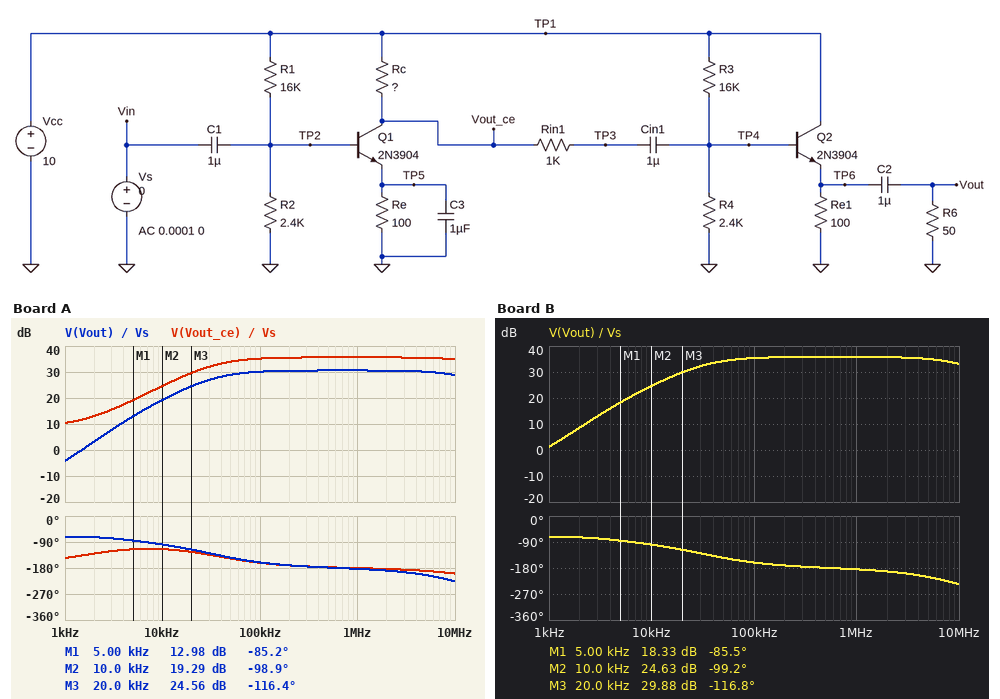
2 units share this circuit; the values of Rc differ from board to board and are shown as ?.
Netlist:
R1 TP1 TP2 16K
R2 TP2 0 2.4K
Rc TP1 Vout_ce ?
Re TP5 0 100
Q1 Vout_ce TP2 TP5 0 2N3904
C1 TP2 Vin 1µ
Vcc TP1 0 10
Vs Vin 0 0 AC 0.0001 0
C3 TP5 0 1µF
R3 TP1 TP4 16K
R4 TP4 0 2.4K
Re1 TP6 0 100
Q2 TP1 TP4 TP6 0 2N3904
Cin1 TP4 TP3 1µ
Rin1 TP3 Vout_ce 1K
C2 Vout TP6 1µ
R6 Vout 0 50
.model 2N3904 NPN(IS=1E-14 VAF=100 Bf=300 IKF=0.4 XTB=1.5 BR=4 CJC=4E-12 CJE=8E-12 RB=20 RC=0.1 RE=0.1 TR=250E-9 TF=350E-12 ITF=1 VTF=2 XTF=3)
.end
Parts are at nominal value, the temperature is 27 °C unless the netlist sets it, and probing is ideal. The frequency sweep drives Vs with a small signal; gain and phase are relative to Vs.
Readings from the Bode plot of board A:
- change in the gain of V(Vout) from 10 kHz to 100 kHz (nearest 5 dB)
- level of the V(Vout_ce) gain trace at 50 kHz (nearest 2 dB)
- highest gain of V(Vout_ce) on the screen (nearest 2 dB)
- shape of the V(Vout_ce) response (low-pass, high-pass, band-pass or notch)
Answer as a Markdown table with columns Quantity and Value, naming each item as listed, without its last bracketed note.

| Quantity | Value |
|---|---|
| change in the gain of V(Vout) from 10 kHz to 100 kHz | 10 dB |
| level of the V(Vout_ce) gain trace at 50 kHz | 34 dB |
| highest gain of V(Vout_ce) on the screen | 36 dB |
| shape of the V(Vout_ce) response | high-pass |
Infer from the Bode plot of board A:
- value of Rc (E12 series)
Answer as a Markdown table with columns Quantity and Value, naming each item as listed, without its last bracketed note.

| Quantity | Value |
|---|---|
| value of Rc | 330 Ω |
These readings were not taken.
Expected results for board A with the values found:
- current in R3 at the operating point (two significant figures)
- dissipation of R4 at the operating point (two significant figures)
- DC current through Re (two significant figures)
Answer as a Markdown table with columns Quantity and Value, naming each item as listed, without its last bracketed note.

| Quantity | Value |
|---|---|
| current in R3 at the operating point | 550 µA |
| dissipation of R4 at the operating point | 670 µW |
| DC current through Re | 5.7 mA |
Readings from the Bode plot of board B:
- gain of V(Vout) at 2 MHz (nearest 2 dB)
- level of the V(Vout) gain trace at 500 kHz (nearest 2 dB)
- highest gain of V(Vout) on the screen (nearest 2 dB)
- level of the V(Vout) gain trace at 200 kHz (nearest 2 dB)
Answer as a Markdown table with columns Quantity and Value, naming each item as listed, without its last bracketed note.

| Quantity | Value |
|---|---|
| gain of V(Vout) at 2 MHz | 36 dB |
| level of the V(Vout) gain trace at 500 kHz | 36 dB |
| highest gain of V(Vout) on the screen | 36 dB |
| level of the V(Vout) gain trace at 200 kHz | 36 dB |
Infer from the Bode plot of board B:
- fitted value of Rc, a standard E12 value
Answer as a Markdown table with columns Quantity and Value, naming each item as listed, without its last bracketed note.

| Quantity | Value |
|---|---|
| fitted value of Rc, a standard E12 value | 680 Ω |
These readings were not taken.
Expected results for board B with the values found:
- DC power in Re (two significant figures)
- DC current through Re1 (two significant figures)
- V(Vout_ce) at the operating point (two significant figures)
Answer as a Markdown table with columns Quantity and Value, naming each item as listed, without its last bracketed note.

| Quantity | Value |
|---|---|
| DC power in Re | 3.2 mW |
| DC current through Re1 | 5.7 mA |
| V(Vout_ce) at the operating point | 6.2 V |
